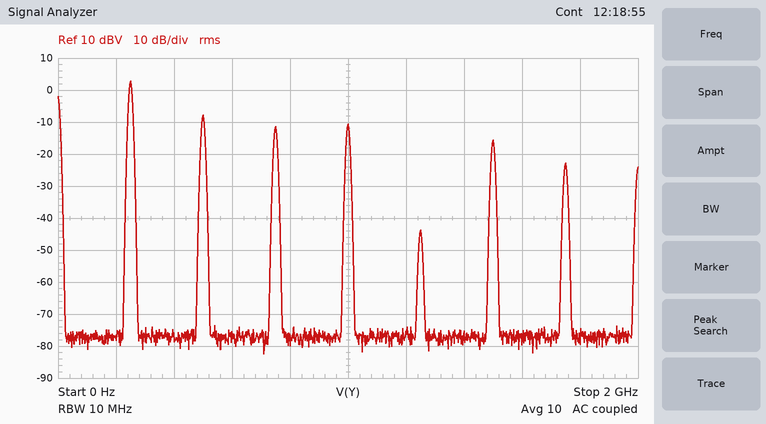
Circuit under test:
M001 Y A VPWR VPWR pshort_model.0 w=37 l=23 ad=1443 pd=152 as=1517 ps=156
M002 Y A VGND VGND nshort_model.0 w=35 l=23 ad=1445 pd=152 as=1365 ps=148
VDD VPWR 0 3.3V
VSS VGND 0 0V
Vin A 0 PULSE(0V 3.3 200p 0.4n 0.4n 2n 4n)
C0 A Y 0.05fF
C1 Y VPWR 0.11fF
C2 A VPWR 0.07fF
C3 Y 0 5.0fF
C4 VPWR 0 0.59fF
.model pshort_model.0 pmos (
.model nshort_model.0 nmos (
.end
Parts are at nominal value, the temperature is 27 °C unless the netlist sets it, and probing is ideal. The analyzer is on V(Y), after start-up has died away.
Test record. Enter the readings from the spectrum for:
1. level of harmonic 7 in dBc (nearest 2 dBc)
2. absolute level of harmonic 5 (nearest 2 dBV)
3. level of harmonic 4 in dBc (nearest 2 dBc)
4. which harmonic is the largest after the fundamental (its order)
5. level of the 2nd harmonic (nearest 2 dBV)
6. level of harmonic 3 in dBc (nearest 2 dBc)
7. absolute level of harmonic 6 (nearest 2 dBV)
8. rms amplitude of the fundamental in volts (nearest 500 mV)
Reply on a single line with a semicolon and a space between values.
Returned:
-26 dBc; -44 dBV; -14 dBc; 2; -8 dBV; -14 dBc; -16 dBV; 1.5 V
